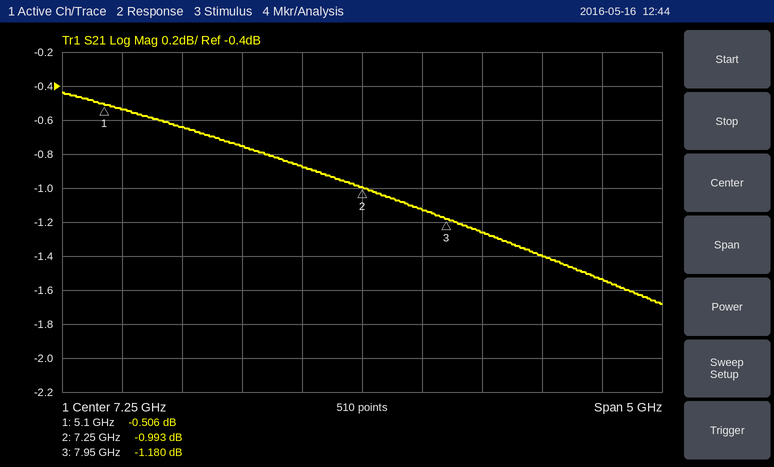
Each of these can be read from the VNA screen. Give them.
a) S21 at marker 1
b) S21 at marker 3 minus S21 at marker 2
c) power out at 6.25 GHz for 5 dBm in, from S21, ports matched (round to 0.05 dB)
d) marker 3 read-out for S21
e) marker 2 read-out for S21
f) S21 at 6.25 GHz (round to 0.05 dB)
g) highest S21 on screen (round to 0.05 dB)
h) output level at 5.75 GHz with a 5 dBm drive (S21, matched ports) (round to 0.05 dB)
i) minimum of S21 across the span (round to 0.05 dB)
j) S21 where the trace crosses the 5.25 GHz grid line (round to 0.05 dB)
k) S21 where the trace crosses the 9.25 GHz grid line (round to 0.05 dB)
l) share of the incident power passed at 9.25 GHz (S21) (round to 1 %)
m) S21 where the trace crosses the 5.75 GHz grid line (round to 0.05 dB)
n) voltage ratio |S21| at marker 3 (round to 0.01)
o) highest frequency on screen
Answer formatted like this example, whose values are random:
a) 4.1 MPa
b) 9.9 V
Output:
a) -0.506 dB
b) -0.187 dB
c) 4.25 dBm
d) -1.180 dB
e) -0.993 dB
f) -0.75 dB
g) -0.45 dB
h) 4.35 dBm
i) -1.70 dB
j) -0.55 dB
k) -1.55 dB
l) 70 %
m) -0.65 dB
n) 0.87
o) 9.75 GHz
